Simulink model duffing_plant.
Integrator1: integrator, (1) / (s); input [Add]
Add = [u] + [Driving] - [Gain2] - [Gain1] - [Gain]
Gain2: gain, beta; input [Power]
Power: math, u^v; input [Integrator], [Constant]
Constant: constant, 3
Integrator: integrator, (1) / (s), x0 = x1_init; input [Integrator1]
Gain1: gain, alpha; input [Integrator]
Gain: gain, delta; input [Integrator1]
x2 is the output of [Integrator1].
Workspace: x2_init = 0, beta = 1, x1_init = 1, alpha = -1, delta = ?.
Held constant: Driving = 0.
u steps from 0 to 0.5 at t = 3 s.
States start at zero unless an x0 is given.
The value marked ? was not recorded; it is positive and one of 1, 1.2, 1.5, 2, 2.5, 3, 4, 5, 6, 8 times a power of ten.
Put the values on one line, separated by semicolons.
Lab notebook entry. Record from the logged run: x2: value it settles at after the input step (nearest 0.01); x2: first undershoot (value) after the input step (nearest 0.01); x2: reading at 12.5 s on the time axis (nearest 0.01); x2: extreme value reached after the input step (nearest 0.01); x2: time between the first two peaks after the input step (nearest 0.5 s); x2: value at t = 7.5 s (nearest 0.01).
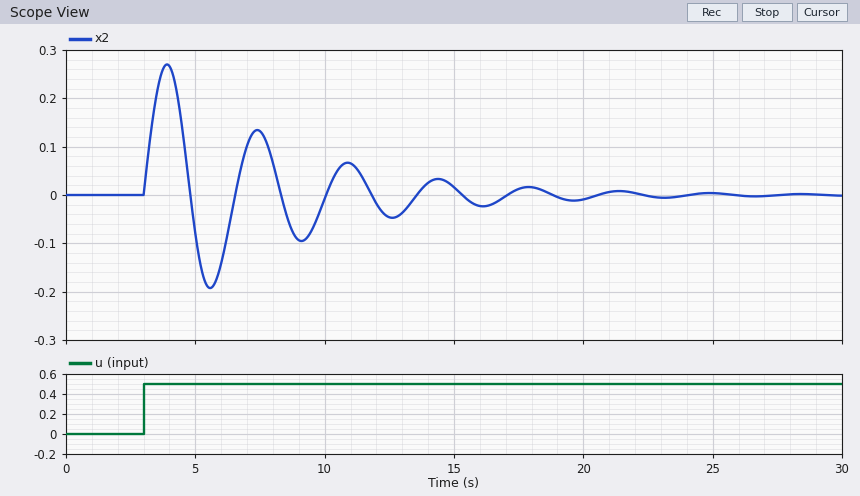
0.00; -0.19; -0.05; 0.27; 3.5 s; 0.13
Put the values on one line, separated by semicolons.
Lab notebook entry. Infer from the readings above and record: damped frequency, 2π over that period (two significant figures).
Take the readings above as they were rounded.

1.8 rad/s
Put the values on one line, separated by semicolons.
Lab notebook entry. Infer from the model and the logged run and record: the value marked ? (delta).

0.4
